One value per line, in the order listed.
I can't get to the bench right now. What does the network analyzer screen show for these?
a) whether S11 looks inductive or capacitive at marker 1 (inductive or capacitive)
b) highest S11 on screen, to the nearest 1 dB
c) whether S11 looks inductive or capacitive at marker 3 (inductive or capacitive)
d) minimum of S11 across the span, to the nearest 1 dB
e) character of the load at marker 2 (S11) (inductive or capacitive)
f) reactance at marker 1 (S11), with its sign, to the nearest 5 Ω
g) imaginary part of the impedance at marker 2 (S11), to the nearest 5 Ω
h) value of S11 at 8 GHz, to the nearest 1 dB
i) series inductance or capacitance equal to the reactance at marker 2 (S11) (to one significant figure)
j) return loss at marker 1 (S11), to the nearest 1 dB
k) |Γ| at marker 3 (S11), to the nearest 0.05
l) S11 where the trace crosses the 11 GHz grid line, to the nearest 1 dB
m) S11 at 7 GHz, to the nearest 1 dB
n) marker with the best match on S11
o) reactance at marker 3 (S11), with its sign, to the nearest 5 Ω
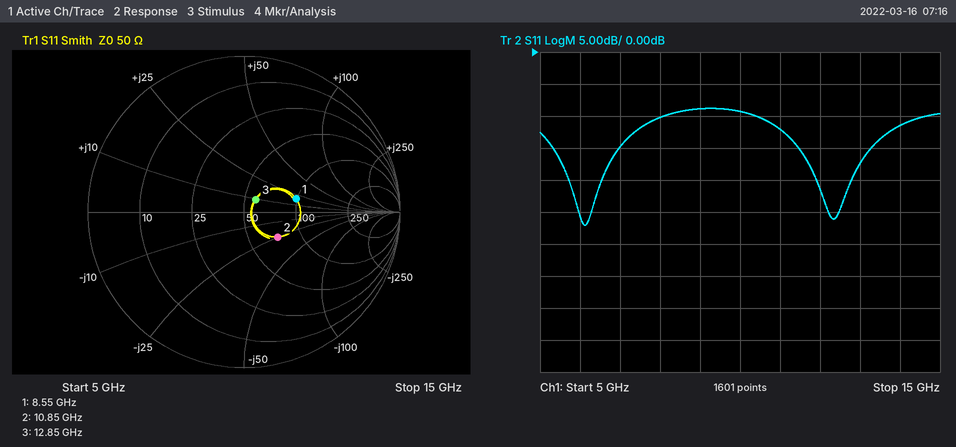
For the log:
inductive
-9 dB
inductive
-27 dB
capacitive
+20 Ω
-25 Ω
-10 dB
600 fF
9 dB
0.10
-12 dB
-15 dB
marker 3
+10 Ω
